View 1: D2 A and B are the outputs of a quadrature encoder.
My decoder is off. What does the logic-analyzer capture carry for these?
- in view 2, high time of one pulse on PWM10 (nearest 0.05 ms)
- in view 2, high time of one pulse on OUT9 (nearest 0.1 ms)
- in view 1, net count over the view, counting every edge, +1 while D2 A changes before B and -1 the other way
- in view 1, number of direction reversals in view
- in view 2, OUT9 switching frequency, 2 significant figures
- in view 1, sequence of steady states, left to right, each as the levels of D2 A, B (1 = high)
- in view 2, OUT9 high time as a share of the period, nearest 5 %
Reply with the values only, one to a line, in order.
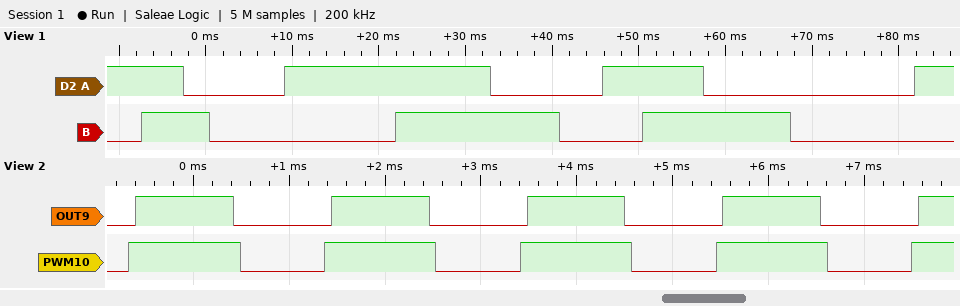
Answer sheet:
1.15 ms
1.0 ms
+12
0
490 Hz
10 11 01 00 10 11 01 00 10 11 01 00 10
50 %
